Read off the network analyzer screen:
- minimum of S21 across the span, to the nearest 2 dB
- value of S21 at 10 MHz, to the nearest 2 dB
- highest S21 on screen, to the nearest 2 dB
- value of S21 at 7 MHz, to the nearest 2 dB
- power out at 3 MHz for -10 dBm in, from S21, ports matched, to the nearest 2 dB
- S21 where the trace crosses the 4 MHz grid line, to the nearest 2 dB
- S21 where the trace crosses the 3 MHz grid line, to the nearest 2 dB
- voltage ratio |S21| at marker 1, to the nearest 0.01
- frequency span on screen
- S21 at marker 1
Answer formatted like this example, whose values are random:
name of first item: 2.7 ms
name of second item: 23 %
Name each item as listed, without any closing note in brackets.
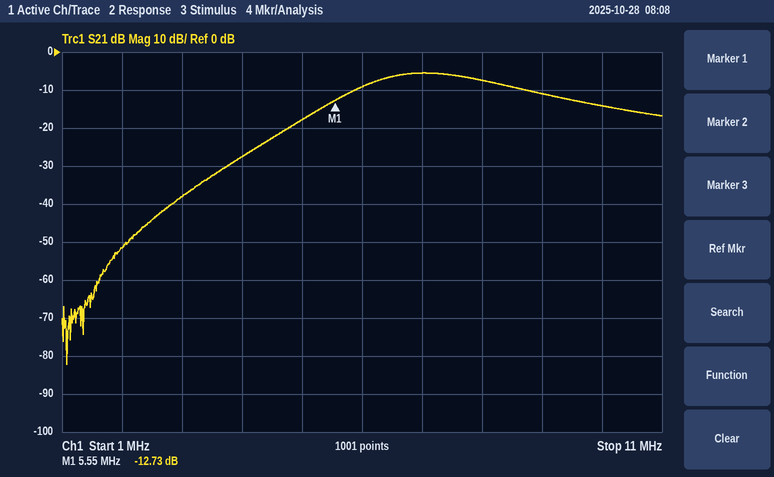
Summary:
minimum of S21 across the span, to the nearest 2 dB: -82 dB
value of S21 at 10 MHz, to the nearest 2 dB: -14 dB
highest S21 on screen, to the nearest 2 dB: -6 dB
value of S21 at 7 MHz, to the nearest 2 dB: -6 dB
power out at 3 MHz for -10 dBm in, from S21, ports matched, to the nearest 2 dB: -48 dBm
S21 where the trace crosses the 4 MHz grid line, to the nearest 2 dB: -28 dB
S21 where the trace crosses the 3 MHz grid line, to the nearest 2 dB: -38 dB
voltage ratio |S21| at marker 1, to the nearest 0.01: 0.23
frequency span on screen: 10 MHz
S21 at marker 1: -12.73 dB
